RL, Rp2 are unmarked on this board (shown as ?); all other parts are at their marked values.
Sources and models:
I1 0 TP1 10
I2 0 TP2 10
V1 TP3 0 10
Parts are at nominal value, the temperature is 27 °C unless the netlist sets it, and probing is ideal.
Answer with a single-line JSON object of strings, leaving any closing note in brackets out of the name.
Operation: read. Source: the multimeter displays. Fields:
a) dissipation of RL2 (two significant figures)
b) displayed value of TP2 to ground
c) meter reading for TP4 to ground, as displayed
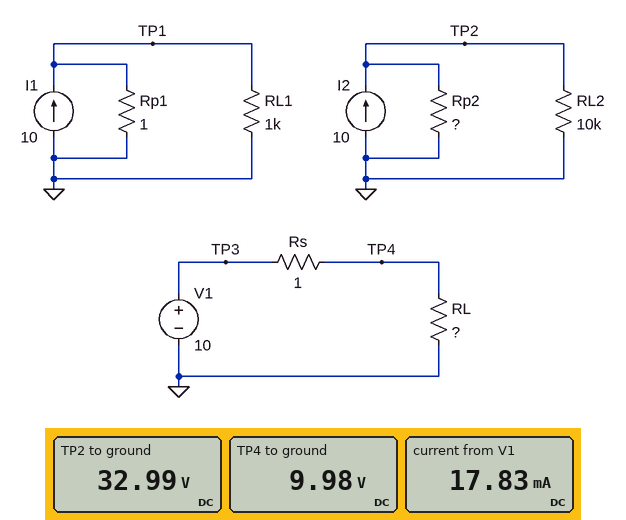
{"dissipation of RL2": "110 mW", "displayed value of TP2 to ground": "32.99 V", "meter reading for TP4 to ground, as displayed": "9.98 V"}
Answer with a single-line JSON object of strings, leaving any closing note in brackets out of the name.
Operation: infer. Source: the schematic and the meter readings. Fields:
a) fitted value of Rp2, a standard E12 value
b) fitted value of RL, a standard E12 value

{"fitted value of Rp2, a standard E12 value": "3.3 Ω", "fitted value of RL, a standard E12 value": "560 Ω"}
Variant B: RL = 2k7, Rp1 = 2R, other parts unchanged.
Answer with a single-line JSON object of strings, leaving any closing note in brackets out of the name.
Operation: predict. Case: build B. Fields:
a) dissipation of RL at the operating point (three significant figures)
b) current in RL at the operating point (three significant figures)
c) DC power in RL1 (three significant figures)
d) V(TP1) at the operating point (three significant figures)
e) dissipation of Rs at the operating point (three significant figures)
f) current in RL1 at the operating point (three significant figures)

{"dissipation of RL at the operating point": "37.0 mW", "current in RL at the operating point": "3.70 mA", "DC power in RL1": "398 mW", "V(TP1) at the operating point": "20.0 V", "dissipation of Rs at the operating point": "13.7 µW", "current in RL1 at the operating point": "20.0 mA"}
